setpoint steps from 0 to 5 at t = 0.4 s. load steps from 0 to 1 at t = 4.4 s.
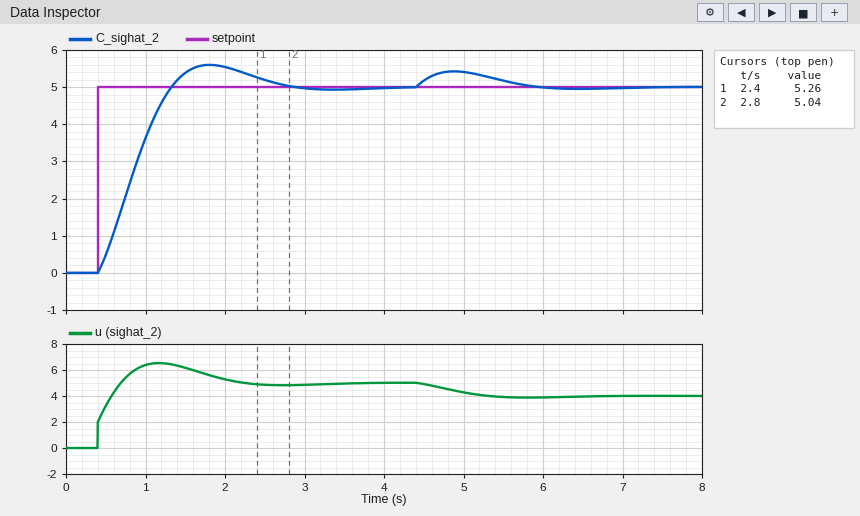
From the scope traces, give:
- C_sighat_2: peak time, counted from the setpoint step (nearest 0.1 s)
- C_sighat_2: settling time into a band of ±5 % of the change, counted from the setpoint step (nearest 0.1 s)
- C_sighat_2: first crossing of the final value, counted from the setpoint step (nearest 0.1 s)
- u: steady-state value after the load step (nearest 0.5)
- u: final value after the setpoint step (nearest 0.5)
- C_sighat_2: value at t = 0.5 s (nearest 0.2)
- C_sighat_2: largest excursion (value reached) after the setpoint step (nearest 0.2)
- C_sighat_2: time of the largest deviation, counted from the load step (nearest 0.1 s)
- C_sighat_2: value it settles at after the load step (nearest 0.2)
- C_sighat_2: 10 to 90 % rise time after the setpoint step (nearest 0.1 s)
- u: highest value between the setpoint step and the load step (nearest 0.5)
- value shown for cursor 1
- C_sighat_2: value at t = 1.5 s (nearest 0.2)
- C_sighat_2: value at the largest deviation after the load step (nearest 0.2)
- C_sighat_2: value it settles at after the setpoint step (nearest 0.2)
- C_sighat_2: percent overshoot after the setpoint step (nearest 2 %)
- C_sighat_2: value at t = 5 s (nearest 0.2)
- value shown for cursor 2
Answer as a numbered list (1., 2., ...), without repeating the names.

1. 1.4 s
2. 2.0 s
3. 0.9 s
4. 4.0
5. 5.0
6. 0.4
7. 5.6
8. 0.5 s
9. 5.0
10. 0.7 s
11. 6.5
12. 5.26
13. 5.4
14. 5.4
15. 5.0
16. 12 %
17. 5.4
18. 5.04
